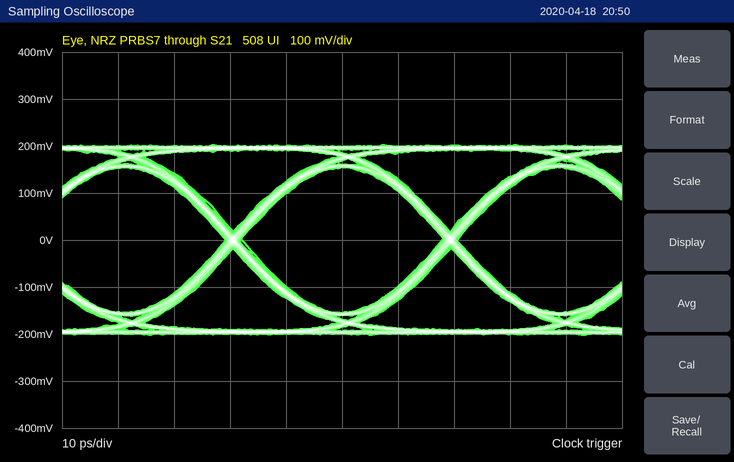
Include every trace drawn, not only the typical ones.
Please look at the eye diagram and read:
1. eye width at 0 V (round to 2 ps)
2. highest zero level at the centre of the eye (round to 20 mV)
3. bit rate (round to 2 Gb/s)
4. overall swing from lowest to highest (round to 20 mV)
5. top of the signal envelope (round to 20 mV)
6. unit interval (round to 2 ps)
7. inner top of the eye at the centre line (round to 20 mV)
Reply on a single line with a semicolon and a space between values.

36 ps; -160 mV; 26 Gb/s; 400 mV; 200 mV; 38 ps; 160 mV
